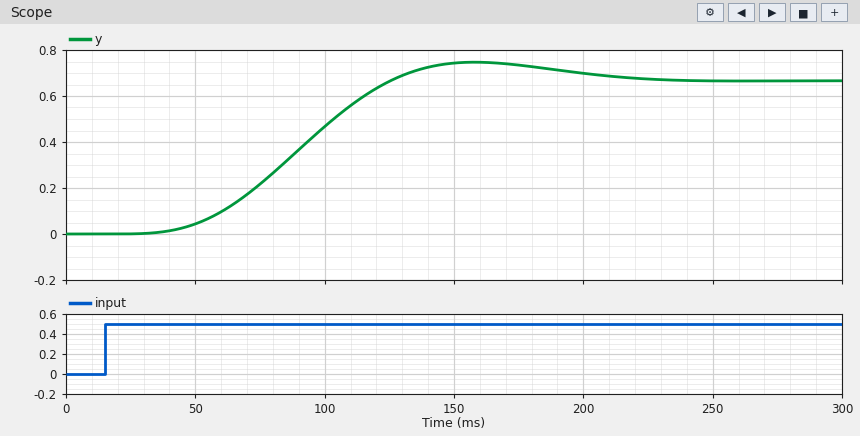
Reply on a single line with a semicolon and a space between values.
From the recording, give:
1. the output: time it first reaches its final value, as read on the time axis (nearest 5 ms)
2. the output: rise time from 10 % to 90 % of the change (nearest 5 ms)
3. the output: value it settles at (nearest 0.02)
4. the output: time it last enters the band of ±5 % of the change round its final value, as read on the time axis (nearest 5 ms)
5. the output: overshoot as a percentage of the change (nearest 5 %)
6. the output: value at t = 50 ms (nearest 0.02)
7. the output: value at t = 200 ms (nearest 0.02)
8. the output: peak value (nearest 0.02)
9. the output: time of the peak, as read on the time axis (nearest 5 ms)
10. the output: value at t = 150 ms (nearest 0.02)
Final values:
125 ms; 60 ms; 0.66; 200 ms; 10 %; 0.04; 0.70; 0.74; 160 ms; 0.74
